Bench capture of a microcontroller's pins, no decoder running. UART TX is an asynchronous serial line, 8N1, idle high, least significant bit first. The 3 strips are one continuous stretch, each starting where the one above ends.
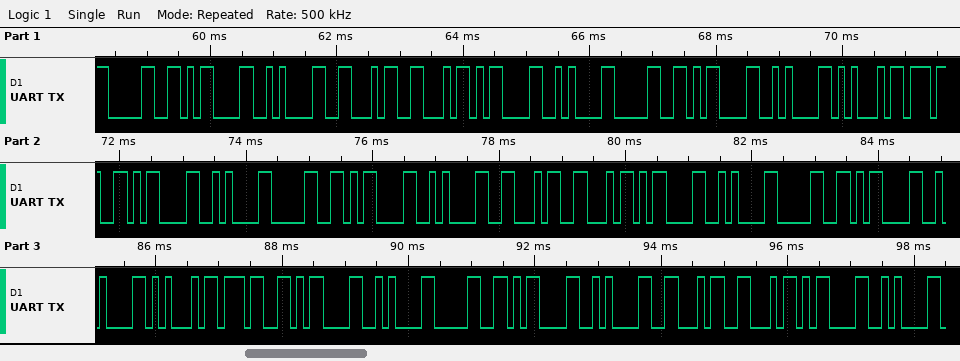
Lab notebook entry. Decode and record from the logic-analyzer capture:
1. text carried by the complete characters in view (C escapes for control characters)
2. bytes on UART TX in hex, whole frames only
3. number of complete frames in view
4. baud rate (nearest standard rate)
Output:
"0\r\nFF\r\n0\r\nE7\r\n0\r\nFF\r\n0\r\nE7\r\n0\r\nFF\r\n"
0x30 0x0D 0x0A 0x46 0x46 0x0D 0x0A 0x30 0x0D 0x0A 0x45 0x37 0x0D 0x0A 0x30 0x0D 0x0A 0x46 0x46 0x0D 0x0A 0x30 0x0D 0x0A 0x45 0x37 0x0D 0x0A 0x30 0x0D 0x0A 0x46 0x46 0x0D 0x0A
35
9600 baud
